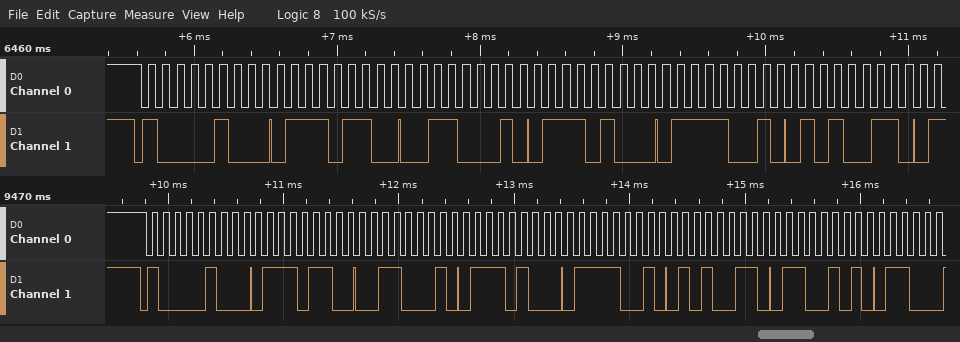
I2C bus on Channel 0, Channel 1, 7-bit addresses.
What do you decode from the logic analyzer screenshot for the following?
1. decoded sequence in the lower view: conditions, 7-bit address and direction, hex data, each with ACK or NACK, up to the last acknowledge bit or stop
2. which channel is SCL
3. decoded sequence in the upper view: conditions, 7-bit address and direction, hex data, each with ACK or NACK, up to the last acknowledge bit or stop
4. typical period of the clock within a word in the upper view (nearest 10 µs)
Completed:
start, address 42 write ACK, 76 ACK, 31 ACK, 74 ACK, 79 ACK, 53 ACK, 65 ACK
Channel 0
start, address 42 write ACK, 76 ACK, 31 ACK, 74 ACK, 79 ACK, 53 ACK
100 µs
